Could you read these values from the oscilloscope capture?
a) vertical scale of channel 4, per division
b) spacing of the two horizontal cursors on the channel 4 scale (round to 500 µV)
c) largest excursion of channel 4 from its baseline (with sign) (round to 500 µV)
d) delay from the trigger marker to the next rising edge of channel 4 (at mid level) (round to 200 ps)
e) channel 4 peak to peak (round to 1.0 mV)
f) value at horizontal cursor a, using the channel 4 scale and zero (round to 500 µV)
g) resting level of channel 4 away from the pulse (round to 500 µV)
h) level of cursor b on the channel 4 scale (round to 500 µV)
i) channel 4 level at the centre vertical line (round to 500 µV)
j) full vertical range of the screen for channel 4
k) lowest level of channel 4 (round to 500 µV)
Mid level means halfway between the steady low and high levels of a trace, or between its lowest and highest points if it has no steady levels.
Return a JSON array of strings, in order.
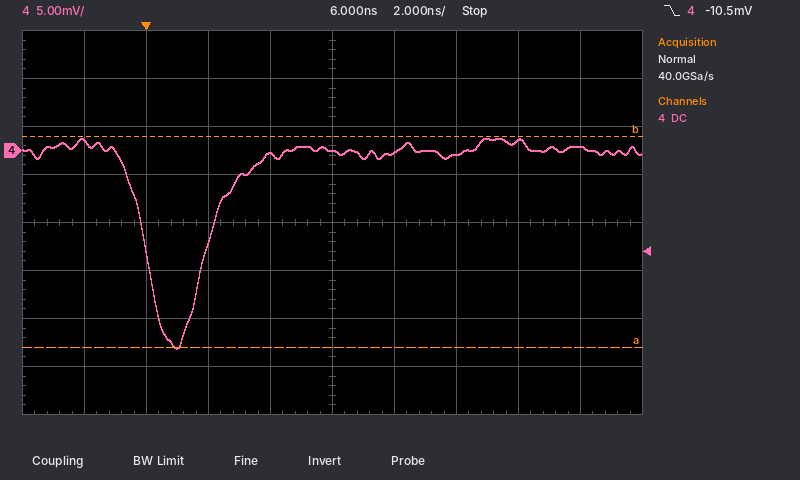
["5 mV", "22.0 mV", "-20.5 mV", "2.0 ns", "22.0 mV", "-20.5 mV", "0.0 mV", "1.5 mV", "0.0 mV", "40 mV", "-20.5 mV"]
